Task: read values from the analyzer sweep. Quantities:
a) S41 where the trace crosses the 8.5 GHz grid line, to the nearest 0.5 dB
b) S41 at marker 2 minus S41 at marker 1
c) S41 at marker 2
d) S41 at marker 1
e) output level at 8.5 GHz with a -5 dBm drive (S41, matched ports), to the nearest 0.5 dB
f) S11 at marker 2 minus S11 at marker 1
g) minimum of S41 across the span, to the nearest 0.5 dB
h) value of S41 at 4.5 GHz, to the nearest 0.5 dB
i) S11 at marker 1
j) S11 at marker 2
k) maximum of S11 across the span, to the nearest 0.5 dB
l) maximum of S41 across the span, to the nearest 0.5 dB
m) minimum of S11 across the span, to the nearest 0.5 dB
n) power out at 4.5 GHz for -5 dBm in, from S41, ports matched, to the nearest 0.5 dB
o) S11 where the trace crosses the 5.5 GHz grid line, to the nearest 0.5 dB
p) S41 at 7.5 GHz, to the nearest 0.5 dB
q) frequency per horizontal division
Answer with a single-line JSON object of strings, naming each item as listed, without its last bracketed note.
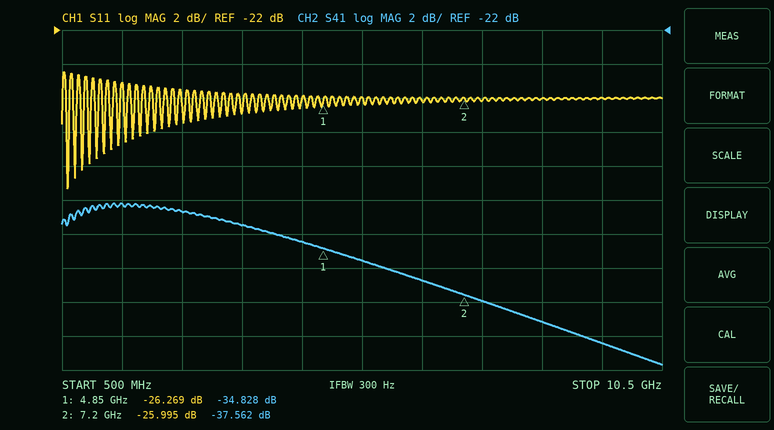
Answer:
{"S41 where the trace crosses the 8.5 GHz grid line, to the nearest 0.5 dB": "-39.0 dB", "S41 at marker 2 minus S41 at marker 1": "-2.734 dB", "S41 at marker 2": "-37.562 dB", "S41 at marker 1": "-34.828 dB", "output level at 8.5 GHz with a -5 dBm drive (S41, matched ports), to the nearest 0.5 dB": "-44.0 dBm", "S11 at marker 2 minus S11 at marker 1": "0.274 dB", "minimum of S41 across the span, to the nearest 0.5 dB": "-41.5 dB", "value of S41 at 4.5 GHz, to the nearest 0.5 dB": "-34.5 dB", "S11 at marker 1": "-26.269 dB", "S11 at marker 2": "-25.995 dB", "maximum of S11 across the span, to the nearest 0.5 dB": "-24.5 dB", "maximum of S41 across the span, to the nearest 0.5 dB": "-32.0 dB", "minimum of S11 across the span, to the nearest 0.5 dB": "-31.5 dB", "power out at 4.5 GHz for -5 dBm in, from S41, ports matched, to the nearest 0.5 dB": "-39.5 dBm", "S11 where the trace crosses the 5.5 GHz grid line, to the nearest 0.5 dB": "-26.0 dB", "S41 at 7.5 GHz, to the nearest 0.5 dB": "-38.0 dB", "frequency per horizontal division": "1 GHz"}
